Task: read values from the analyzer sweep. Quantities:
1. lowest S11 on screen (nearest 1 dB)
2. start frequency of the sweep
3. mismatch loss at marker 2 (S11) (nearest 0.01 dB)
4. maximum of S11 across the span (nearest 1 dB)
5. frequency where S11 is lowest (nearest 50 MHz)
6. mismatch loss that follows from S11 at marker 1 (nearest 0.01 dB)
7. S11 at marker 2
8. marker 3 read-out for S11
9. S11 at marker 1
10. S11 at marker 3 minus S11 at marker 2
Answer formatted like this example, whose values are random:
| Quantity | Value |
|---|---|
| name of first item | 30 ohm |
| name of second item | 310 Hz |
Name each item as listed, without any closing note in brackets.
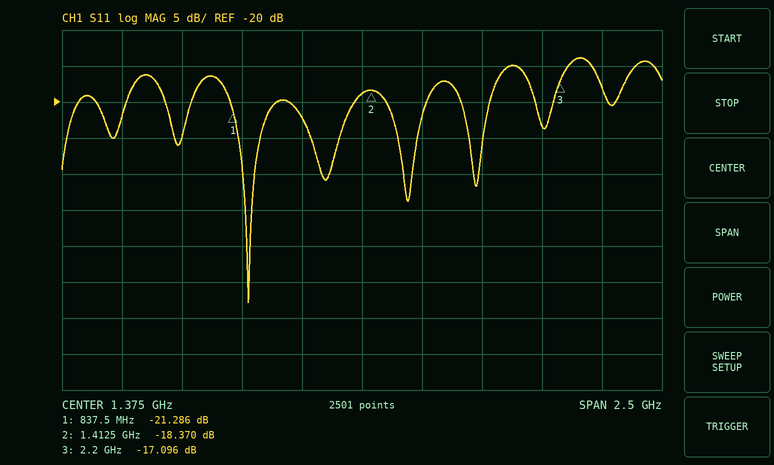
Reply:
| Quantity | Value |
|---|---|
| lowest S11 on screen | -48 dB |
| start frequency of the sweep | 125 MHz |
| mismatch loss at marker 2 (S11) | 0.06 dB |
| maximum of S11 across the span | -14 dB |
| frequency where S11 is lowest | 900 MHz |
| mismatch loss that follows from S11 at marker 1 | 0.03 dB |
| S11 at marker 2 | -18.370 dB |
| marker 3 read-out for S11 | -17.096 dB |
| S11 at marker 1 | -21.286 dB |
| S11 at marker 3 minus S11 at marker 2 | 1.274 dB |
